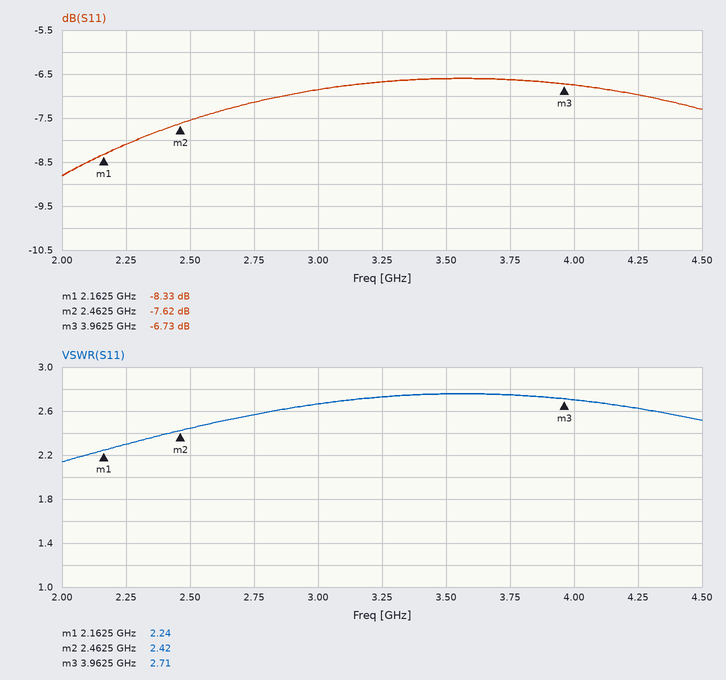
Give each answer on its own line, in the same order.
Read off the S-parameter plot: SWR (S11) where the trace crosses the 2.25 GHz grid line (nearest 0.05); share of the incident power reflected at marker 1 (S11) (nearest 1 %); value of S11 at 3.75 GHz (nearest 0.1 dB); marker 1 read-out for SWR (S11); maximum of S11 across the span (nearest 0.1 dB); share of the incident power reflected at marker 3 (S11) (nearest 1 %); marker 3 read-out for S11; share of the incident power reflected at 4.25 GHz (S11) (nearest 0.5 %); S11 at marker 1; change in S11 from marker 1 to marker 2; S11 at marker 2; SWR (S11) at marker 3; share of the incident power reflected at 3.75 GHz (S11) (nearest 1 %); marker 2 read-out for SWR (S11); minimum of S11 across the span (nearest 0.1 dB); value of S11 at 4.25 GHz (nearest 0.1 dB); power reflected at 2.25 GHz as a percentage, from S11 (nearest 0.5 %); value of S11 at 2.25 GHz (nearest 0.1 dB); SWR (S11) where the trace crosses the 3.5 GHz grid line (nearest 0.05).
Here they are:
2.30
15 %
-6.6 dB
2.24
-6.6 dB
21 %
-6.73 dB
20.0 %
-8.33 dB
0.71 dB
-7.62 dB
2.71
22 %
2.42
-8.8 dB
-7.0 dB
15.5 %
-8.1 dB
2.75
